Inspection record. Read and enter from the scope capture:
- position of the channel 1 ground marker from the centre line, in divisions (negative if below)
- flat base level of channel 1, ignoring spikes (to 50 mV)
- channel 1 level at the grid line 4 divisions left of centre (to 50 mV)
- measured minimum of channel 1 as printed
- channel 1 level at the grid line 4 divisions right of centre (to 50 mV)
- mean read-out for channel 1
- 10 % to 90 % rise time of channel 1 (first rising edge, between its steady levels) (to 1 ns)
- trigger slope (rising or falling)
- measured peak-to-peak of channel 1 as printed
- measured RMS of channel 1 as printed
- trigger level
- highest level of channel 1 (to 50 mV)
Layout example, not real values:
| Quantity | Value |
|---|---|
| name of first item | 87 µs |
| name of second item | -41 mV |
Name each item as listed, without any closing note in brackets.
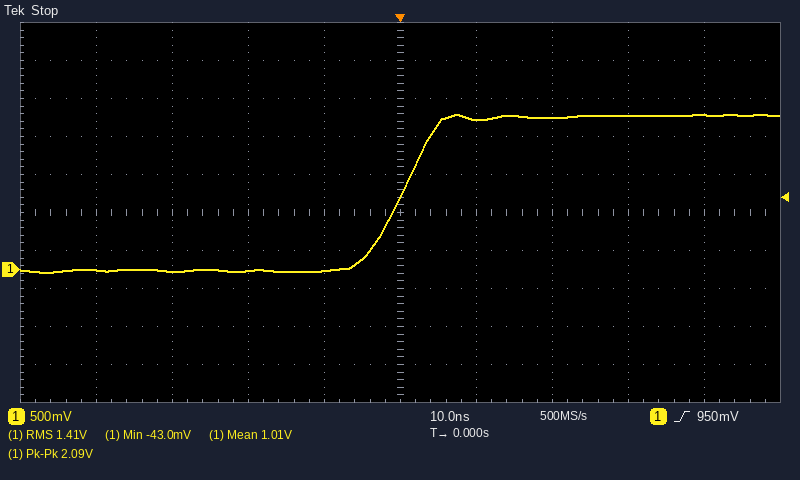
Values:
| Quantity | Value |
|---|---|
| position of the channel 1 ground marker from the centre line, in divisions | -1.5 div |
| flat base level of channel 1, ignoring spikes | 0 mV |
| channel 1 level at the grid line 4 divisions left of centre | 0 mV |
| measured minimum of channel 1 as printed | -43.0 mV |
| channel 1 level at the grid line 4 divisions right of centre | 2.05 V |
| mean read-out for channel 1 | 1.01 V |
| 10 % to 90 % rise time of channel 1 (first rising edge, between its steady levels) | 9 ns |
| trigger slope | rising |
| measured peak-to-peak of channel 1 as printed | 2.09 V |
| measured RMS of channel 1 as printed | 1.41 V |
| trigger level | 950 mV |
| highest level of channel 1 | 2.05 V |
